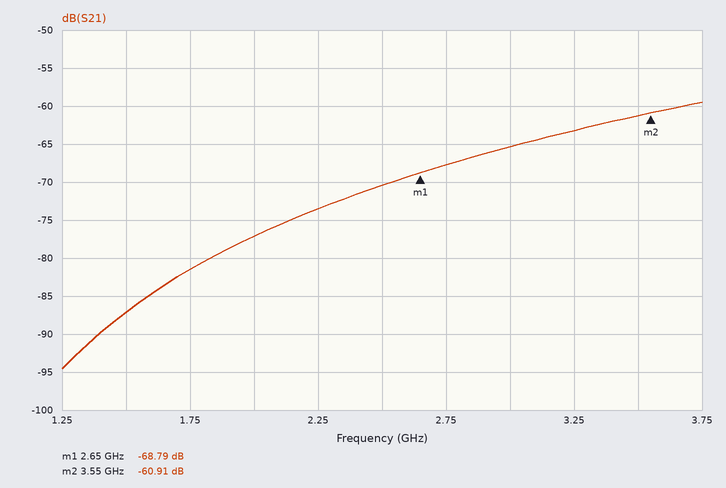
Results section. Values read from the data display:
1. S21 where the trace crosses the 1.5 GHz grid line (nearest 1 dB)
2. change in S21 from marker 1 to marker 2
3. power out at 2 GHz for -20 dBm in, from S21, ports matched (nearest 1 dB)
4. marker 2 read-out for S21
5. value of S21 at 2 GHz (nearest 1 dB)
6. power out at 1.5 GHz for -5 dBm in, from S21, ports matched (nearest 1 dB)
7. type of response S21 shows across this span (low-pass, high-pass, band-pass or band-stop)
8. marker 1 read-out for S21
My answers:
-87 dB
7.88 dB
-97 dBm
-60.91 dB
-77 dB
-92 dBm
high-pass
-68.79 dB
